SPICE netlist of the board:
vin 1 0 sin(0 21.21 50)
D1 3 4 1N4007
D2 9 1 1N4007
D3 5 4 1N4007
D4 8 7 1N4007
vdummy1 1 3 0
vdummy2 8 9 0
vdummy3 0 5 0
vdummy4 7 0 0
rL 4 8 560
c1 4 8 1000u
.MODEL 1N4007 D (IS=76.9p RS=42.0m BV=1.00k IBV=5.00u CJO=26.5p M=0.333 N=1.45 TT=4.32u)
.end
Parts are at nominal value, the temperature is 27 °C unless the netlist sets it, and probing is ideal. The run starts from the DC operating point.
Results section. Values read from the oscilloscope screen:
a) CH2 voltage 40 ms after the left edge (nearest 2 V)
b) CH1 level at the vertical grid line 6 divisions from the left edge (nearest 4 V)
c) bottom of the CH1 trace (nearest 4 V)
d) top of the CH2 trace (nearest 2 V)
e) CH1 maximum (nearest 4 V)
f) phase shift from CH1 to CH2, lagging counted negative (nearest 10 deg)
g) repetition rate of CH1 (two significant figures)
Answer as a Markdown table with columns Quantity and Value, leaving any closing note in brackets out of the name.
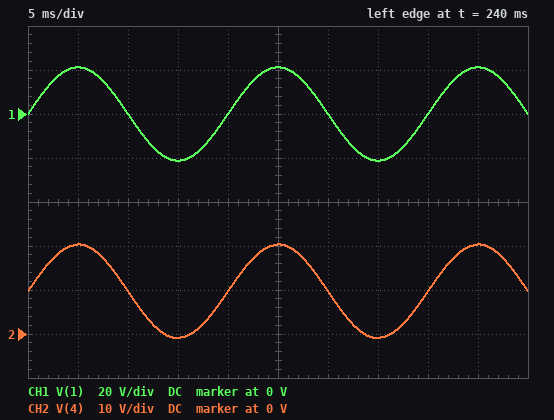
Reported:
| Quantity | Value |
|---|---|
| CH2 voltage 40 ms after the left edge | 10 V |
| CH1 level at the vertical grid line 6 divisions from the left edge | 0 V |
| bottom of the CH1 trace | -20 V |
| top of the CH2 trace | 20 V |
| CH1 maximum | 20 V |
| phase shift from CH1 to CH2, lagging counted negative | 0 deg |
| repetition rate of CH1 | 50 Hz |
